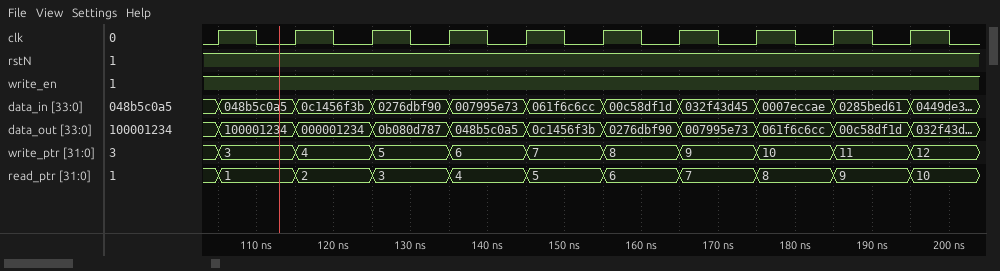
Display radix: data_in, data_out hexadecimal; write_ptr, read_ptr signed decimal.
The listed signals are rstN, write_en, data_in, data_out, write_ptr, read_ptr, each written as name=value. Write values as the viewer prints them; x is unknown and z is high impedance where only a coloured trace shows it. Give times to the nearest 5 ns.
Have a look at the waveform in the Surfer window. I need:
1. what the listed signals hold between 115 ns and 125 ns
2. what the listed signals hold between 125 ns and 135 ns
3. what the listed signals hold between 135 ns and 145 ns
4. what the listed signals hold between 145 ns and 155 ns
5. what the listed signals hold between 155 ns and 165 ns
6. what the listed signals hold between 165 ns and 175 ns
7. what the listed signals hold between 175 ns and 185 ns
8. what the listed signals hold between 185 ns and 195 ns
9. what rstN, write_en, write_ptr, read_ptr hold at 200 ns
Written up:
rstN=1, write_en=1, data_in=0c1456f3b, data_out=000001234, write_ptr=4, read_ptr=2
rstN=1, write_en=1, data_in=0276dbf90, data_out=0b080d787, write_ptr=5, read_ptr=3
rstN=1, write_en=1, data_in=007995e73, data_out=048b5c0a5, write_ptr=6, read_ptr=4
rstN=1, write_en=1, data_in=061f6c6cc, data_out=0c1456f3b, write_ptr=7, read_ptr=5
rstN=1, write_en=1, data_in=00c58df1d, data_out=0276dbf90, write_ptr=8, read_ptr=6
rstN=1, write_en=1, data_in=032f43d45, data_out=007995e73, write_ptr=9, read_ptr=7
rstN=1, write_en=1, data_in=0007eccae, data_out=061f6c6cc, write_ptr=10, read_ptr=8
rstN=1, write_en=1, data_in=0285bed61, data_out=00c58df1d, write_ptr=11, read_ptr=9
rstN=1, write_en=1, write_ptr=12, read_ptr=10
